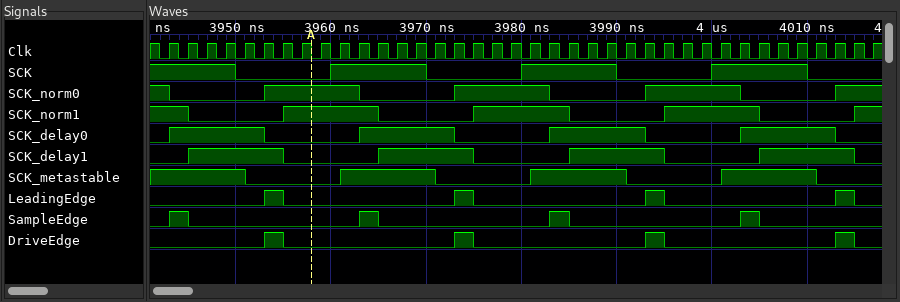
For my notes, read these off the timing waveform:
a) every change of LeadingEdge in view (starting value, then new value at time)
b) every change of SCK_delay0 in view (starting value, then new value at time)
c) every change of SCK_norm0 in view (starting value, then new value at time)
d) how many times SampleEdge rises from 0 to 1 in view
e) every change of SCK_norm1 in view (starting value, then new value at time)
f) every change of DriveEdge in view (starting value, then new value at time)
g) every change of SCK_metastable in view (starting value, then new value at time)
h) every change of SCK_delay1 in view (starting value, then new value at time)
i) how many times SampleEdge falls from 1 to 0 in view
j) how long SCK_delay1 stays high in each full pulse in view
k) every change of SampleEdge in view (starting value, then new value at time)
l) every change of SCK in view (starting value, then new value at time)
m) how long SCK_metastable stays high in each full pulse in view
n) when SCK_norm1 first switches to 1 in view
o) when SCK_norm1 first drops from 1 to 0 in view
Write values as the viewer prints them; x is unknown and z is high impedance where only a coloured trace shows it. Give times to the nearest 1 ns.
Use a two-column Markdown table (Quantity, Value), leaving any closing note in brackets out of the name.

| Quantity | Value |
|---|---|
| every change of LeadingEdge in view | 0, 1 at 3953 ns, 0 at 3955 ns, 1 at 3973 ns, 0 at 3975 ns, 1 at 3993 ns, 0 at 3995 ns, 1 at 4013 ns, 0 at 4015 ns |
| every change of SCK_delay0 in view | 0, 1 at 3943 ns, 0 at 3953 ns, 1 at 3963 ns, 0 at 3973 ns, 1 at 3983 ns, 0 at 3993 ns, 1 at 4003 ns, 0 at 4013 ns |
| every change of SCK_norm0 in view | 1, 0 at 3943 ns, 1 at 3953 ns, 0 at 3963 ns, 1 at 3973 ns, 0 at 3983 ns, 1 at 3993 ns, 0 at 4003 ns, 1 at 4013 ns |
| how many times SampleEdge rises from 0 to 1 in view | 4 |
| every change of SCK_norm1 in view | 1, 0 at 3945 ns, 1 at 3955 ns, 0 at 3965 ns, 1 at 3975 ns, 0 at 3985 ns, 1 at 3995 ns, 0 at 4005 ns, 1 at 4015 ns |
| every change of DriveEdge in view | 0, 1 at 3953 ns, 0 at 3955 ns, 1 at 3973 ns, 0 at 3975 ns, 1 at 3993 ns, 0 at 3995 ns, 1 at 4013 ns, 0 at 4015 ns |
| every change of SCK_metastable in view | 1, 0 at 3951 ns, 1 at 3961 ns, 0 at 3971 ns, 1 at 3981 ns, 0 at 3991 ns, 1 at 4001 ns, 0 at 4011 ns |
| every change of SCK_delay1 in view | 0, 1 at 3945 ns, 0 at 3955 ns, 1 at 3965 ns, 0 at 3975 ns, 1 at 3985 ns, 0 at 3995 ns, 1 at 4005 ns, 0 at 4015 ns |
| how many times SampleEdge falls from 1 to 0 in view | 4 |
| how long SCK_delay1 stays high in each full pulse in view | 10 ns, 10 ns, 10 ns, 10 ns |
| every change of SampleEdge in view | 0, 1 at 3943 ns, 0 at 3945 ns, 1 at 3963 ns, 0 at 3965 ns, 1 at 3983 ns, 0 at 3985 ns, 1 at 4003 ns, 0 at 4005 ns |
| every change of SCK in view | 1, 0 at 3950 ns, 1 at 3960 ns, 0 at 3970 ns, 1 at 3980 ns, 0 at 3990 ns, 1 at 4000 ns, 0 at 4010 ns |
| how long SCK_metastable stays high in each full pulse in view | 10 ns, 10 ns, 10 ns |
| when SCK_norm1 first switches to 1 in view | 3955 ns |
| when SCK_norm1 first drops from 1 to 0 in view | 3945 ns |
